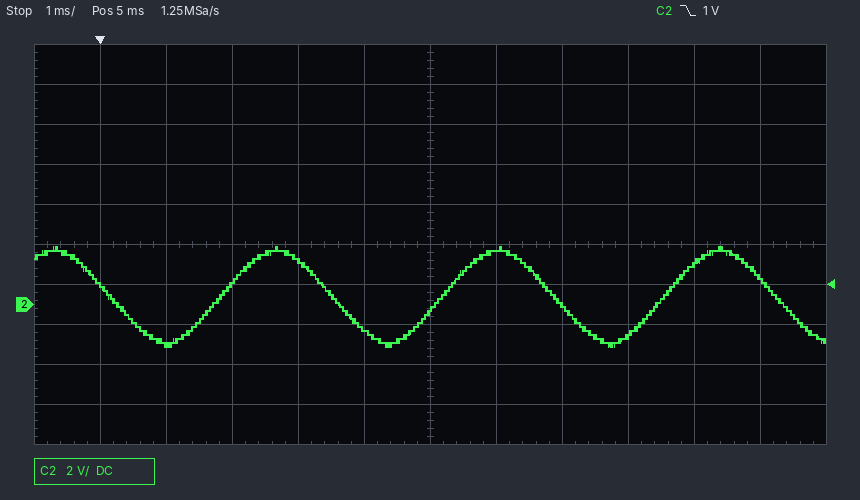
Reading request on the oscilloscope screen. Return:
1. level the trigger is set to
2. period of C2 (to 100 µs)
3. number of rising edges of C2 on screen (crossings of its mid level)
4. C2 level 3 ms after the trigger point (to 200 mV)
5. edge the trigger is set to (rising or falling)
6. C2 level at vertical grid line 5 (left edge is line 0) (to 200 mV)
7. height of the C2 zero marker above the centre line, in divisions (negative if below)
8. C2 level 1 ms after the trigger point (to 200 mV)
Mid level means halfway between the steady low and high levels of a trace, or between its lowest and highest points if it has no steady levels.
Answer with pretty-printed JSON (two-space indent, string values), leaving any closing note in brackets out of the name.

{
  "level the trigger is set to": "1 V",
  "period of C2": "3.4 ms",
  "number of rising edges of C2 on screen": "3",
  "C2 level 3 ms after the trigger point": "2.2 V",
  "edge the trigger is set to": "falling",
  "C2 level at vertical grid line 5 (left edge is line 0)": "-1.2 V",
  "height of the C2 zero marker above the centre line, in divisions": "-1.5 div",
  "C2 level 1 ms after the trigger point": "-2.0 V"
}
